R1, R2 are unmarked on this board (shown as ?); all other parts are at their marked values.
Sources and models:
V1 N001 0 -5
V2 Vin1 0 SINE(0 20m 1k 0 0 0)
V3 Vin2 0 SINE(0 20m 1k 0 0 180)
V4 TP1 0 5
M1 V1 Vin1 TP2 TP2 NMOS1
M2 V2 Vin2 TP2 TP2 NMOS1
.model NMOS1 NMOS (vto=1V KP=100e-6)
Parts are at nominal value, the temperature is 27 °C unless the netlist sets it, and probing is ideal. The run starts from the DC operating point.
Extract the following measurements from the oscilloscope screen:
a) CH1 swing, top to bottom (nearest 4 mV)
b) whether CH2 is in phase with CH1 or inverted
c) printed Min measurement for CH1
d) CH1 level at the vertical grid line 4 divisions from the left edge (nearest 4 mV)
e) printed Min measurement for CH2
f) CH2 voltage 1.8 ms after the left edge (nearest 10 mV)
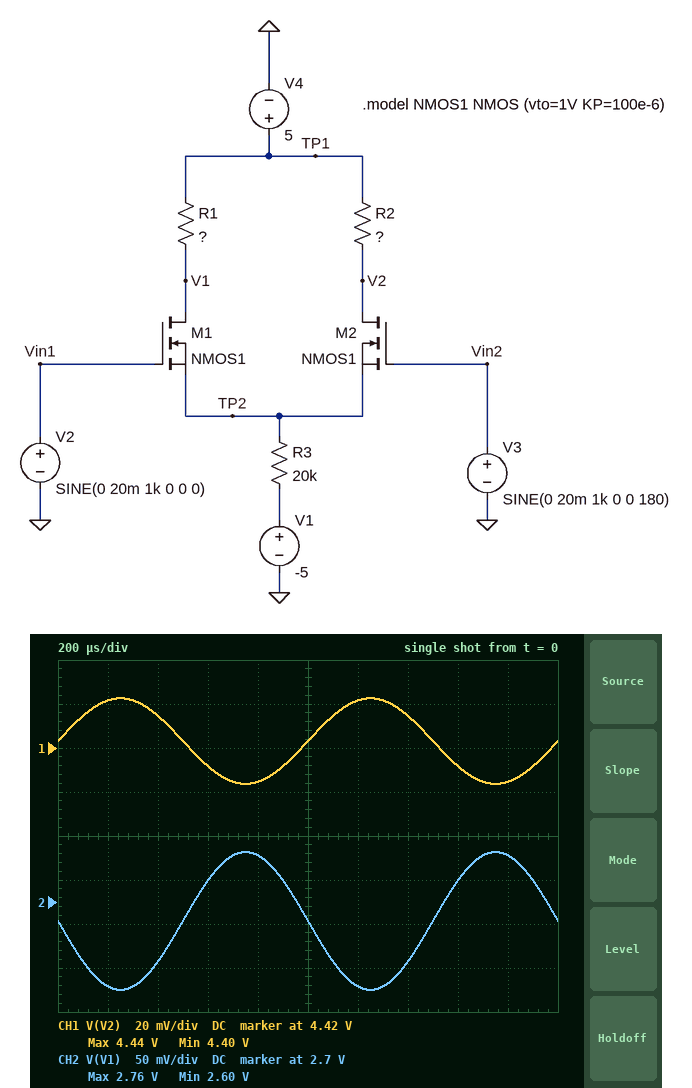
40 mV
inverted
4.40 V
4.404 V
2.60 V
2.75 V
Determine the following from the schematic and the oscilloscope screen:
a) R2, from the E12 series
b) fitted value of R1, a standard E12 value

8.2 kΩ
33 kΩ
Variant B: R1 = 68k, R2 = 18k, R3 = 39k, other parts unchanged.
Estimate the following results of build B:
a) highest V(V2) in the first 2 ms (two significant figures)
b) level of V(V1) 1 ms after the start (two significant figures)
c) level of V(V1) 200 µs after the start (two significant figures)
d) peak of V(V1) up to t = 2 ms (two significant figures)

4.3 V
2.3 V
2.2 V
2.4 V
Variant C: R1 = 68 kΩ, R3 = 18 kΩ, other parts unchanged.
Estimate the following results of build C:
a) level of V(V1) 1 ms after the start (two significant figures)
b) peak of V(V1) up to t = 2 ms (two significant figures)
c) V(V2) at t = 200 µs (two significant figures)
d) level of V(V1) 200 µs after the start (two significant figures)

-220 mV
-48 mV
4.4 V
-380 mV
